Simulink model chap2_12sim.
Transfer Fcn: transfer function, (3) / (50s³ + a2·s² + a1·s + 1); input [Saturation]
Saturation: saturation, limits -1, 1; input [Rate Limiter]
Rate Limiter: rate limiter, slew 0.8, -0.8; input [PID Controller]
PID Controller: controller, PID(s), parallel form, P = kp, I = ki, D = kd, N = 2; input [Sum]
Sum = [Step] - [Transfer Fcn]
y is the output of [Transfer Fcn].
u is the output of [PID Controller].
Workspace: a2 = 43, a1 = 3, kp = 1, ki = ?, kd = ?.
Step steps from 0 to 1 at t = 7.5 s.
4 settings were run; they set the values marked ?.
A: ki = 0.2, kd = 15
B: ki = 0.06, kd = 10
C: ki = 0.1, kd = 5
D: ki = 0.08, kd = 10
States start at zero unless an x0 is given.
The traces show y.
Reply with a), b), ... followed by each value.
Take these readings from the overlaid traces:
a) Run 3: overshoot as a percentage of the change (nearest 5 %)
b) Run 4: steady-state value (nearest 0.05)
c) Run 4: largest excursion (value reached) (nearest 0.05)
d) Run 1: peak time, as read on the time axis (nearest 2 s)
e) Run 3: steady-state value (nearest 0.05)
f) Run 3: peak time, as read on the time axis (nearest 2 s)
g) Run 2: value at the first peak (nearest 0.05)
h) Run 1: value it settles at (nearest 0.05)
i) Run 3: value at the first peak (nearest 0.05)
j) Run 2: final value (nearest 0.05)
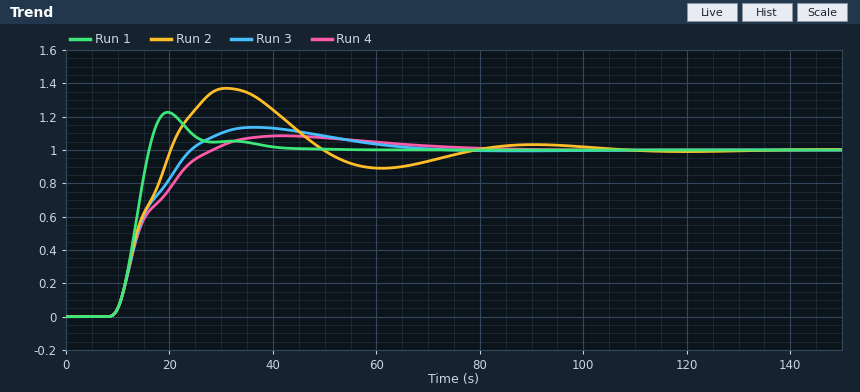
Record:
a) 15 %
b) 1.00
c) 1.10
d) 20 s
e) 1.00
f) 36 s
g) 1.35
h) 1.00
i) 1.15
j) 1.00
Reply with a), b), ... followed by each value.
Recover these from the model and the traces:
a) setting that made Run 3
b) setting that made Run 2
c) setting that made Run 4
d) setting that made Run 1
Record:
a) D
b) A
c) B
d) C
